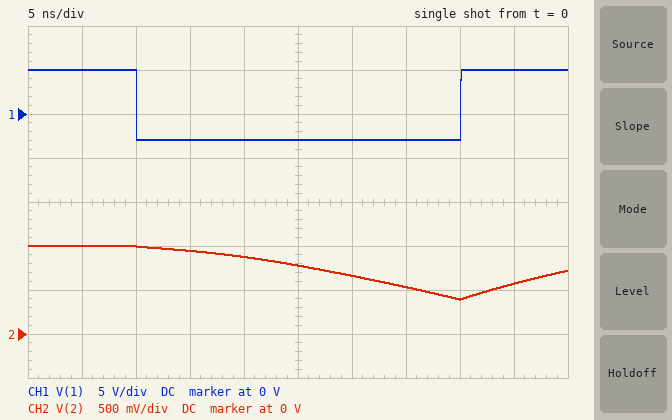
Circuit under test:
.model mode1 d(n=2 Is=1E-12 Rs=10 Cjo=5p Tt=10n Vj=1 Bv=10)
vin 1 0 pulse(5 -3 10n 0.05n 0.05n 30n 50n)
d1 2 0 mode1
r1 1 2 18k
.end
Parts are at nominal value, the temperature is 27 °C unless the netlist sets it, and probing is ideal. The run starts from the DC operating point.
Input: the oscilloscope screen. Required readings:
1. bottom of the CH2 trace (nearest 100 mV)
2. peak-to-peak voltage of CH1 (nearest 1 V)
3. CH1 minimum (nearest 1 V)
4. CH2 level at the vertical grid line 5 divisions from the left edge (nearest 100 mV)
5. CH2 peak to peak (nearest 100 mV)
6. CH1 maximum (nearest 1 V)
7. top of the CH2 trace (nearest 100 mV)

400 mV
8 V
-3 V
800 mV
600 mV
5 V
1.0 V
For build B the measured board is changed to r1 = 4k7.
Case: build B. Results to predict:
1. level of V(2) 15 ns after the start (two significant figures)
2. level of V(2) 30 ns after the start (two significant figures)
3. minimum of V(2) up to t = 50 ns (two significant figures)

990 mV
-390 mV
-1.6 V
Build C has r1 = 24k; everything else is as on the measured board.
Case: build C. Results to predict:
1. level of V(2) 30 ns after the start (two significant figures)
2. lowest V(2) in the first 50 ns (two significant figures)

720 mV
530 mV
